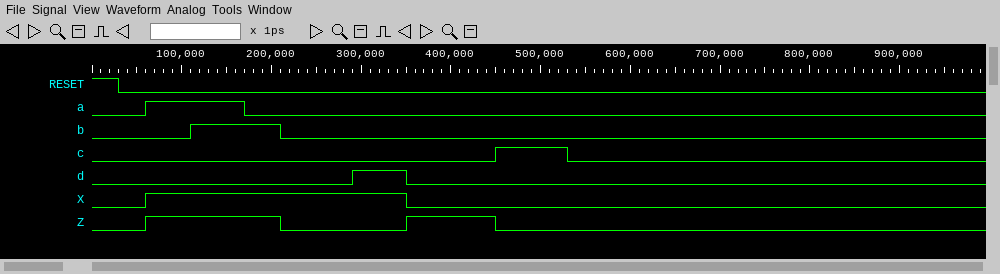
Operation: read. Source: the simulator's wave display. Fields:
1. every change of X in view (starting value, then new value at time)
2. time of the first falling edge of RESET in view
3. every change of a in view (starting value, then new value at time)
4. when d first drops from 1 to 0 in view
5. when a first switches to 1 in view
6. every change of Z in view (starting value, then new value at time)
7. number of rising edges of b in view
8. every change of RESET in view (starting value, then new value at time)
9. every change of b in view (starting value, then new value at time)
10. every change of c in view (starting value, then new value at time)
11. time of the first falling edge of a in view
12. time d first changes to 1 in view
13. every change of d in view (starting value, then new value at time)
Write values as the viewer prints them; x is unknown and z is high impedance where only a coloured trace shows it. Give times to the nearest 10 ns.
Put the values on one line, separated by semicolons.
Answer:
0, 1 at 60 ns, 0 at 350 ns; 30 ns; 0, 1 at 60 ns, 0 at 170 ns; 350 ns; 60 ns; 0, 1 at 60 ns, 0 at 210 ns, 1 at 350 ns, 0 at 450 ns; 1; 1, 0 at 30 ns; 0, 1 at 110 ns, 0 at 210 ns; 0, 1 at 450 ns, 0 at 530 ns; 170 ns; 290 ns; 0, 1 at 290 ns, 0 at 350 ns
